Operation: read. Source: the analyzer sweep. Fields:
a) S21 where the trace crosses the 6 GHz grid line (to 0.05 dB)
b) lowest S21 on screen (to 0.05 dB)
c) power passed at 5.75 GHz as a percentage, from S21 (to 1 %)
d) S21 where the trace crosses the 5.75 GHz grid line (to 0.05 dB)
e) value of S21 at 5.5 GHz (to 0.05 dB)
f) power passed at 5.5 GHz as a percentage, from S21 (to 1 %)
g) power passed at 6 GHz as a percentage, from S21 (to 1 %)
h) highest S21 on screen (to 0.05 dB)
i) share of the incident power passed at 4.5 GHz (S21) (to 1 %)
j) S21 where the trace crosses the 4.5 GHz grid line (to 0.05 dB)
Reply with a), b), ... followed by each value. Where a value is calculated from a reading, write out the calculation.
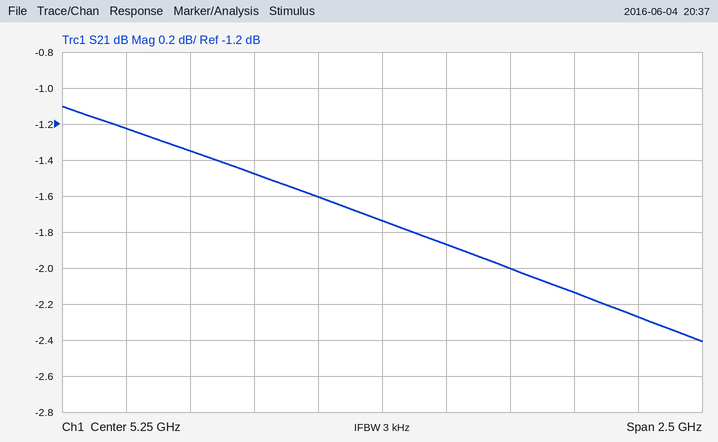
a) -2.15 dB
b) -2.40 dB
c) 10^(-2/10) ≈ 63 %
d) -2.00 dB
e) -1.85 dB
f) 10^(-1.85/10) ≈ 65 %
g) 10^(-2.15/10) ≈ 61 %
h) -1.10 dB
i) 10^(-1.35/10) ≈ 73 %
j) -1.35 dB
